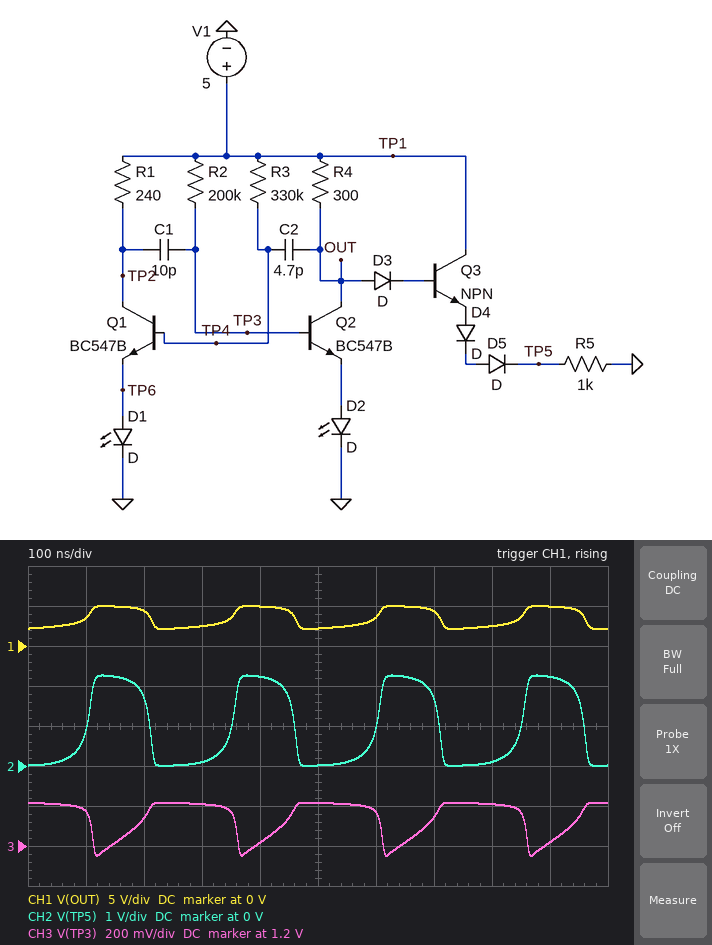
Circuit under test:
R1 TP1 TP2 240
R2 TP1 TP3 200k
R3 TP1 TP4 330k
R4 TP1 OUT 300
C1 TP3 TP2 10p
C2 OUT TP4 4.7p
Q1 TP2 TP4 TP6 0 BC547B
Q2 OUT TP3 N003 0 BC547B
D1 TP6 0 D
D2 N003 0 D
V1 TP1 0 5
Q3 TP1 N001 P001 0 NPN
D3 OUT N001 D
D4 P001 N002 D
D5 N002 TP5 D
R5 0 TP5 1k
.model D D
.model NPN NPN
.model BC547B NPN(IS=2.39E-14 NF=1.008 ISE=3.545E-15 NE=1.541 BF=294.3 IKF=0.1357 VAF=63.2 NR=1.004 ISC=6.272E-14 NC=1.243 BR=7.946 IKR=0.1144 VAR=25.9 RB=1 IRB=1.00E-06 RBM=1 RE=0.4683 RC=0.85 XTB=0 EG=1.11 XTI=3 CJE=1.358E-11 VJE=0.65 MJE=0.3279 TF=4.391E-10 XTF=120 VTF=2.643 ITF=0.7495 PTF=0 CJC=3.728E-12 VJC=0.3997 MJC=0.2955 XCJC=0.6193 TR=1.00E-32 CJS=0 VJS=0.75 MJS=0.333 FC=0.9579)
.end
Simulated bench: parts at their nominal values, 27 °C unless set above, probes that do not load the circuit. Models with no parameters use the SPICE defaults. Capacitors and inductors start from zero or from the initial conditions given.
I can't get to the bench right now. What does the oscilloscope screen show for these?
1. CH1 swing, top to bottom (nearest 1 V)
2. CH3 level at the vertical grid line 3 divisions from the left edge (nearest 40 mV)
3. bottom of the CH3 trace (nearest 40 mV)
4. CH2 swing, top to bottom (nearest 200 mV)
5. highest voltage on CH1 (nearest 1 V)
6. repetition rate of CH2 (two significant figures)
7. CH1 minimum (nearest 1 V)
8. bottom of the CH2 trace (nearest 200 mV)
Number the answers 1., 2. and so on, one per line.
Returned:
1. 3 V
2. 1.40 V
3. 1.16 V
4. 2.2 V
5. 5 V
6. 4.0 MHz
7. 2 V
8. 0 V
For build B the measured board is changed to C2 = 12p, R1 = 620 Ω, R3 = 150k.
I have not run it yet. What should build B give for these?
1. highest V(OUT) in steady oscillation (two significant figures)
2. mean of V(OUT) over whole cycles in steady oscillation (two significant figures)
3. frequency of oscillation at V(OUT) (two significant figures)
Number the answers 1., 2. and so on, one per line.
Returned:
1. 5.0 V
2. 3.9 V
3. 660 kHz
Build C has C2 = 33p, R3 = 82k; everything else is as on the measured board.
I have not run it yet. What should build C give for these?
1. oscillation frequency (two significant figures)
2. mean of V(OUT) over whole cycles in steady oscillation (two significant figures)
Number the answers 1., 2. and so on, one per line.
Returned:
1. 710 kHz
2. 3.4 V
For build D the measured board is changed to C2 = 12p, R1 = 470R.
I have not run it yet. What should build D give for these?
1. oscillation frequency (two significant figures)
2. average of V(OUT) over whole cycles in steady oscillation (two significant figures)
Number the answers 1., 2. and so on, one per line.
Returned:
1. 810 kHz
2. 3.4 V
